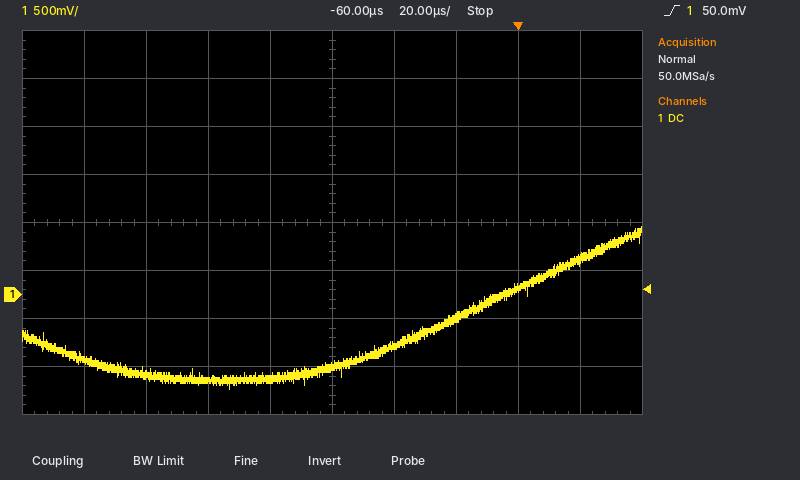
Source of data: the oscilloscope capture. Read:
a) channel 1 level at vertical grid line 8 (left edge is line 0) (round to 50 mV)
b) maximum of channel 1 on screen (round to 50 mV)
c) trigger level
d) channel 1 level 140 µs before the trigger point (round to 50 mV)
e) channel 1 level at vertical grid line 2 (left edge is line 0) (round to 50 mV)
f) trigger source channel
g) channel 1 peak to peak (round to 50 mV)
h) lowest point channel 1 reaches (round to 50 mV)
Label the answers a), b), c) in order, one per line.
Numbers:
a) 50 mV
b) 700 mV
c) 50.0 mV
d) -700 mV
e) -850 mV
f) channel 1
g) 1.70 V
h) -1.00 V
